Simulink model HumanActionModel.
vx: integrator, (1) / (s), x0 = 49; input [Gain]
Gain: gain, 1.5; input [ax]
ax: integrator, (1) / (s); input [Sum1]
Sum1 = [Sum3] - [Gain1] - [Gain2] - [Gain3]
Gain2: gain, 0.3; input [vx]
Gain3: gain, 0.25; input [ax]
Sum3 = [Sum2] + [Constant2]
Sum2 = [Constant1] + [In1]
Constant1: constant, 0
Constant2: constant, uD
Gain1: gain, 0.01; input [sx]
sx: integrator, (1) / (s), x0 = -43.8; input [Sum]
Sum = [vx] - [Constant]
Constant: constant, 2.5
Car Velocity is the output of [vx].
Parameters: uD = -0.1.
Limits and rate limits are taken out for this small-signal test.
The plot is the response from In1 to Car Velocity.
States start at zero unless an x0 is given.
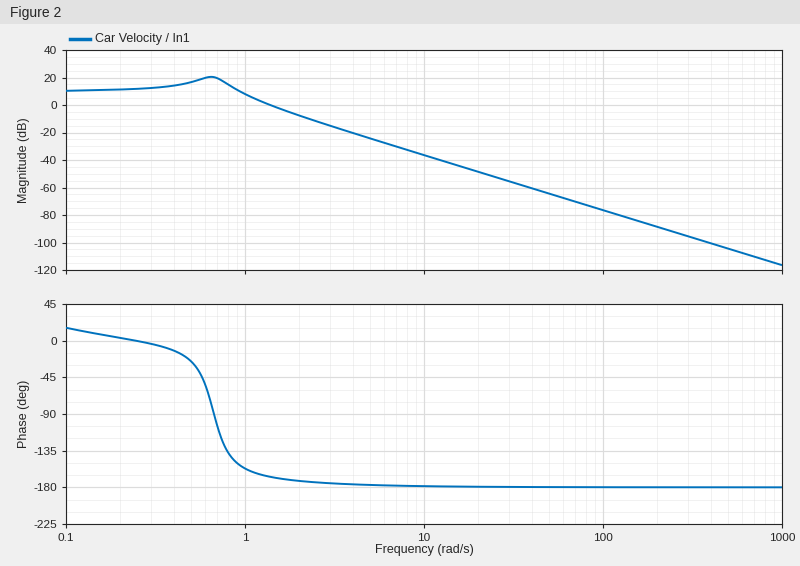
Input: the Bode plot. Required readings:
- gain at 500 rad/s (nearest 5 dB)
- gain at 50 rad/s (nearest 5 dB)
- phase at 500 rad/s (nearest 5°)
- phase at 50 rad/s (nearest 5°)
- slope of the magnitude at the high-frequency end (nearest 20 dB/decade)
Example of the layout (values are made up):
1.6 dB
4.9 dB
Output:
-105 dB
-65 dB
-180°
-180°
-40 dB/decade
